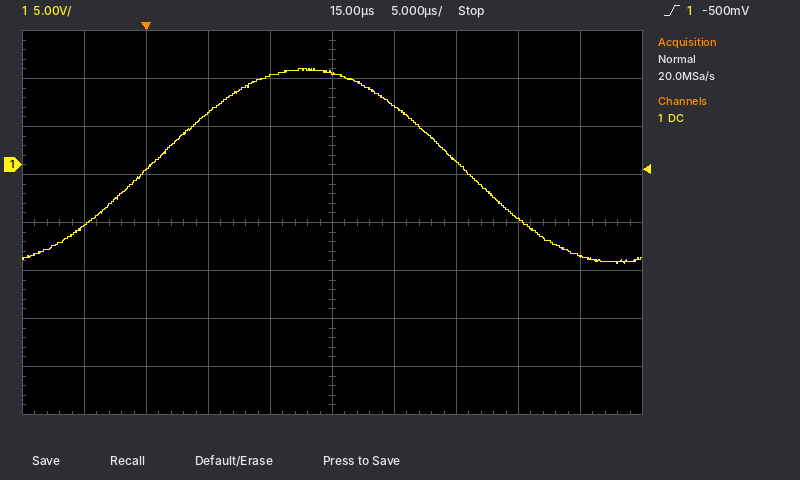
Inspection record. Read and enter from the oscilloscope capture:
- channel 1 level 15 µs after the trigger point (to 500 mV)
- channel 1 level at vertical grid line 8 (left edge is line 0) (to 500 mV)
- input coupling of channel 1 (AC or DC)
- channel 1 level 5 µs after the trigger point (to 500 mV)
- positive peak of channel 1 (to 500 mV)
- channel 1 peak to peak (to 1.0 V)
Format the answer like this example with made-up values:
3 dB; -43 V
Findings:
9.5 V; -5.5 V; DC; 5.5 V; 10.0 V; 20.0 V
